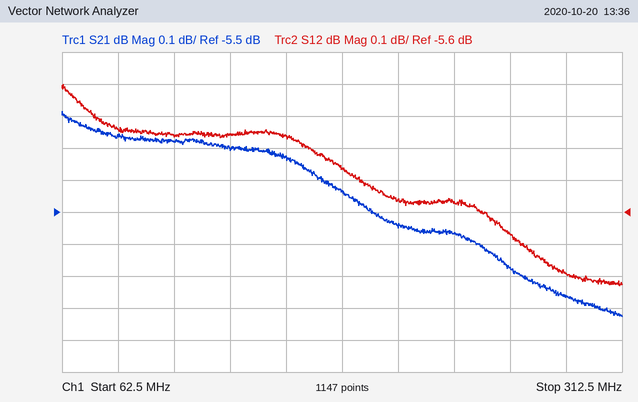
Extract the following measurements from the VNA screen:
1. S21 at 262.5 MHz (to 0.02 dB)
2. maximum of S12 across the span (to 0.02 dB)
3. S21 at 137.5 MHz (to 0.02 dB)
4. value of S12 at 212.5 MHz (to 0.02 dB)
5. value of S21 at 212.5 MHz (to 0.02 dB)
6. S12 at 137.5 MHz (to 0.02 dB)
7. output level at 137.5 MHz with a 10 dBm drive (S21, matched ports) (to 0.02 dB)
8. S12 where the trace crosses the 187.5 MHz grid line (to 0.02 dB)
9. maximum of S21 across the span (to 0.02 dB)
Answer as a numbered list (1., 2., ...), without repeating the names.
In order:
1. -5.68 dB
2. -5.20 dB
3. -5.30 dB
4. -5.56 dB
5. -5.54 dB
6. -5.36 dB
7. 4.70 dBm
8. -5.46 dB
9. -5.18 dB
